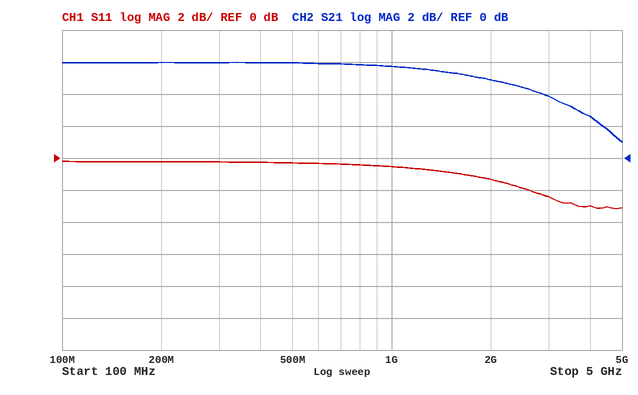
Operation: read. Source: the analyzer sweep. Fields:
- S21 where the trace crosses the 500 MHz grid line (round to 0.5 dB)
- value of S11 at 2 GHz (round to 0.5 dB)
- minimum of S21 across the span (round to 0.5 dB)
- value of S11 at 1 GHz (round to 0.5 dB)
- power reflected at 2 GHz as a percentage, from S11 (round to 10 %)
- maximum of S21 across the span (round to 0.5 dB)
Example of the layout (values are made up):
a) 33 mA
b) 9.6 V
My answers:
a) 6.0 dB
b) -1.5 dB
c) 1.0 dB
d) -0.5 dB
e) 70 %
f) 6.0 dB
